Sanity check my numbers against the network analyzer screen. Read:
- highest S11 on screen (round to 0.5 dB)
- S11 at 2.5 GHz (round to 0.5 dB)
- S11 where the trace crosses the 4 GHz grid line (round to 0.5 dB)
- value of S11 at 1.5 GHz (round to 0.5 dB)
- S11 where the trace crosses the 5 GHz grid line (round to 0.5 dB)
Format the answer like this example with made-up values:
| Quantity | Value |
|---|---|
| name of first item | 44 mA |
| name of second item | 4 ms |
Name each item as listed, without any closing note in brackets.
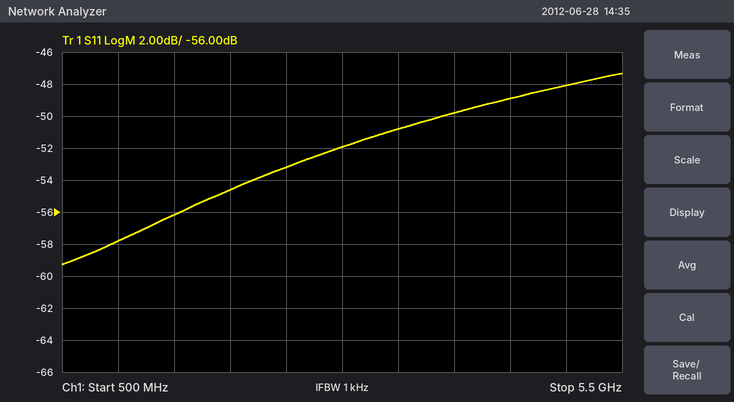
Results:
| Quantity | Value |
|---|---|
| highest S11 on screen | -47.5 dB |
| S11 at 2.5 GHz | -53.0 dB |
| S11 where the trace crosses the 4 GHz grid line | -50.0 dB |
| value of S11 at 1.5 GHz | -56.0 dB |
| S11 where the trace crosses the 5 GHz grid line | -48.0 dB |
